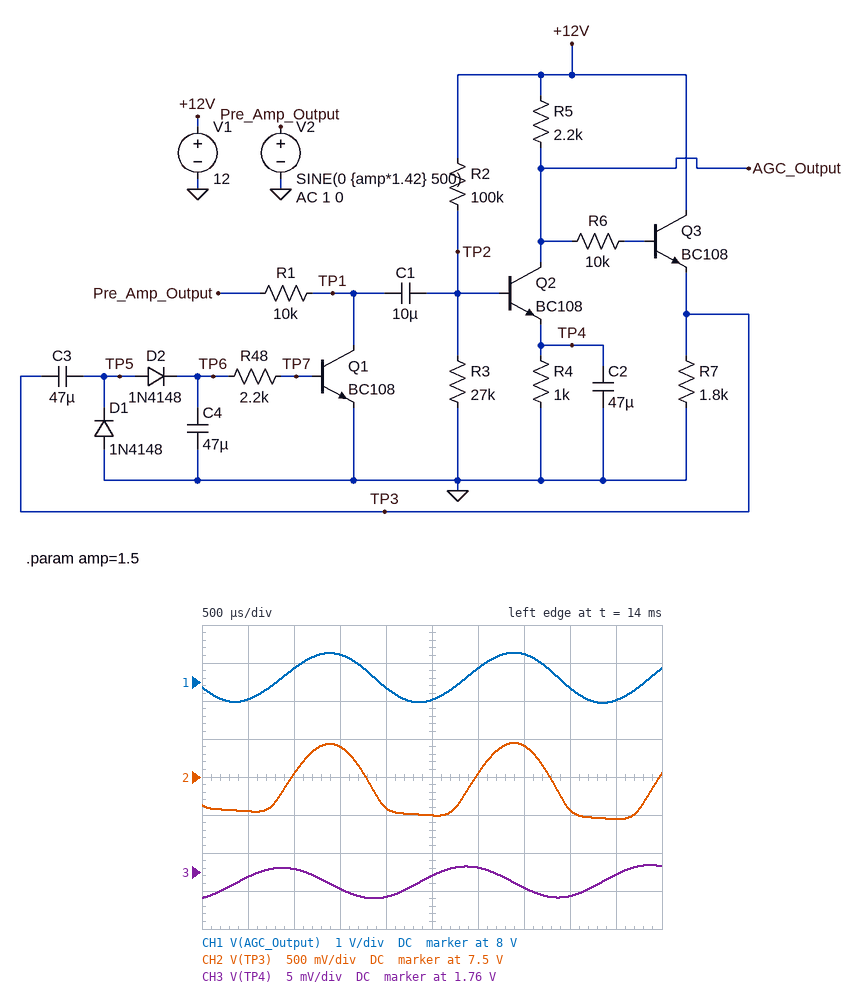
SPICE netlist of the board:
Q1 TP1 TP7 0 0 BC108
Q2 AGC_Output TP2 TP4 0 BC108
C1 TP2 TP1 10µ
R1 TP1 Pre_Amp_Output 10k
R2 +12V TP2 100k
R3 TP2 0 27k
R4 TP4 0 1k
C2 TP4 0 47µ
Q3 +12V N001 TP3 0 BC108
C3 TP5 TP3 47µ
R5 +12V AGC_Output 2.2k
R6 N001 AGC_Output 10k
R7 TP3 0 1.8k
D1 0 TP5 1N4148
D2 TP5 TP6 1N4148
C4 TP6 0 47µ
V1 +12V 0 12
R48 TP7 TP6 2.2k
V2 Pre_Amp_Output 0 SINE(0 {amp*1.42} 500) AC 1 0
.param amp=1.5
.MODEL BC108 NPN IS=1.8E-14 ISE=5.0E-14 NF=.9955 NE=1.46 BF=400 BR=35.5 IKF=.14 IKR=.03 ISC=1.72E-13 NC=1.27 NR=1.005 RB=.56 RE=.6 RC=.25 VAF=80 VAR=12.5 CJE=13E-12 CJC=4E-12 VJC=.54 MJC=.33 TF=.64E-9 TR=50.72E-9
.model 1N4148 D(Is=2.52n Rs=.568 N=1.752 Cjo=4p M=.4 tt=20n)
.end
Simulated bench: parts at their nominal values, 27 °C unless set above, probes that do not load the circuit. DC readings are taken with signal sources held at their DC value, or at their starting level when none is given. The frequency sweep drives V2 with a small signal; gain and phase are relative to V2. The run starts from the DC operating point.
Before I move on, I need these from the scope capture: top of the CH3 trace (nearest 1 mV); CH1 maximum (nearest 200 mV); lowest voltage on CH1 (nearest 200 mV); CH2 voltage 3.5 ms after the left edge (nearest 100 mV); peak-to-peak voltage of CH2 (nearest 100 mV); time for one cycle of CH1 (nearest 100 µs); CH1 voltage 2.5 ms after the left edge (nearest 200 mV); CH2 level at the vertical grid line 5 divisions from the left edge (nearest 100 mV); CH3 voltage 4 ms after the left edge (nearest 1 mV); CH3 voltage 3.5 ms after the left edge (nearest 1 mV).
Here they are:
1.761 V
8.8 V
7.4 V
7.9 V
1.0 V
2.0 ms
7.6 V
7.0 V
1.757 V
1.758 V
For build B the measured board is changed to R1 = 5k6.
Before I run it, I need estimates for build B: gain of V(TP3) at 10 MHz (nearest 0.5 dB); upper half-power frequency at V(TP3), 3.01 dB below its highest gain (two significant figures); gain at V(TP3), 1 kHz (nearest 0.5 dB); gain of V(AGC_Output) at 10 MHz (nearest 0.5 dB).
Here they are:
-3.0 dB
220 kHz
35.0 dB
1.5 dB
